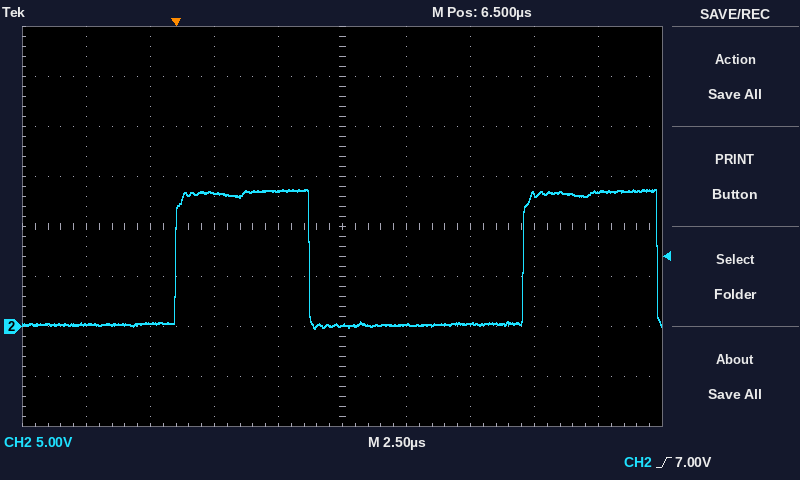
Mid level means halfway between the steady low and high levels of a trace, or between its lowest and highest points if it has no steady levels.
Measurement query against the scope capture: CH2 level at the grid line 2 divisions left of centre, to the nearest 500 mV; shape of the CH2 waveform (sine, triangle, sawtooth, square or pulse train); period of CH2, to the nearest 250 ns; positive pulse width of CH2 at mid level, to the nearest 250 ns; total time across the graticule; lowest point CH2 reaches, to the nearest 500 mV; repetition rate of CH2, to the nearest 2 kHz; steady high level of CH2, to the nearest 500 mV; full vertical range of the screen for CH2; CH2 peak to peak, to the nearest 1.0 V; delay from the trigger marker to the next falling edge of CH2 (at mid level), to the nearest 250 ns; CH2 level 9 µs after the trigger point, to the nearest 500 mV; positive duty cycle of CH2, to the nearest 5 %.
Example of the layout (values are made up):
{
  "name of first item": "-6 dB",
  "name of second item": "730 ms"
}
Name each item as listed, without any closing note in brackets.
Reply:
{
  "CH2 level at the grid line 2 divisions left of centre, to the nearest 500 mV": "13.5 V",
  "shape of the CH2 waveform": "pulse train",
  "period of CH2, to the nearest 250 ns": "13.50 µs",
  "positive pulse width of CH2 at mid level, to the nearest 250 ns": "5.25 µs",
  "total time across the graticule": "25 µs",
  "lowest point CH2 reaches, to the nearest 500 mV": "0.0 V",
  "repetition rate of CH2, to the nearest 2 kHz": "74 kHz",
  "steady high level of CH2, to the nearest 500 mV": "13.5 V",
  "full vertical range of the screen for CH2": "40 V",
  "CH2 peak to peak, to the nearest 1.0 V": "14.0 V",
  "delay from the trigger marker to the next falling edge of CH2 (at mid level), to the nearest 250 ns": "5.25 µs",
  "CH2 level 9 µs after the trigger point, to the nearest 500 mV": "0.0 V",
  "positive duty cycle of CH2, to the nearest 5 %": "40 %"
}
